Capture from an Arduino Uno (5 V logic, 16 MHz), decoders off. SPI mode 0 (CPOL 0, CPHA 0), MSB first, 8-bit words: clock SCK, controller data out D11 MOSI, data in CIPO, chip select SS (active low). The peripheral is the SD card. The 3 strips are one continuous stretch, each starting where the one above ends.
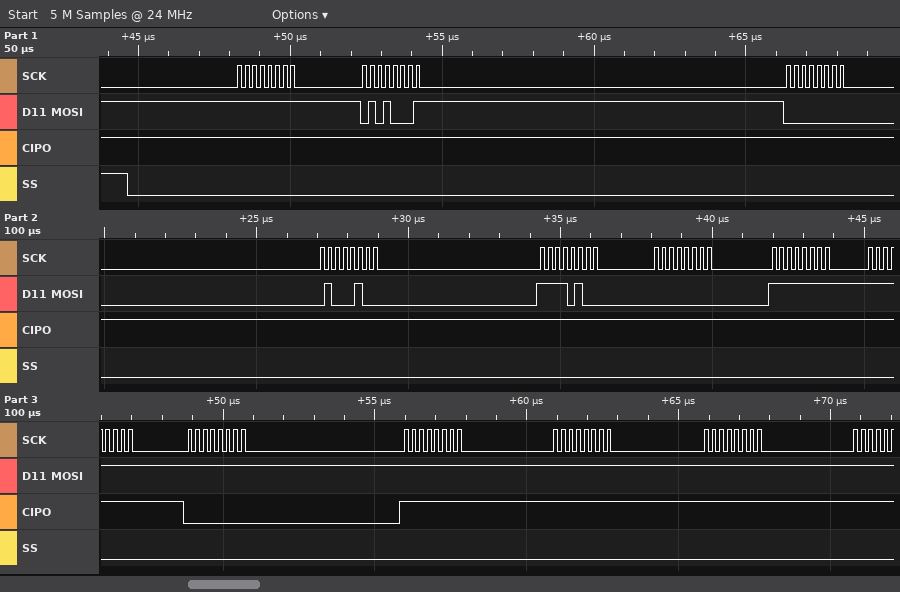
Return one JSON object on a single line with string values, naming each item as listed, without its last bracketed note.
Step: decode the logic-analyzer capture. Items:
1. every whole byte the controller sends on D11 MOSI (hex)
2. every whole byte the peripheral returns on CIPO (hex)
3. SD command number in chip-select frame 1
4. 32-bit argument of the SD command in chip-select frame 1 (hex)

{"every whole byte the controller sends on D11 MOSI": "FF 51 00 44 F4 00 FF FF FF FF FF FF", "every whole byte the peripheral returns on CIPO": "FF FF FF FF FF FF FF FF 00 FF FF FF", "SD command number in chip-select frame 1": "CMD17", "32-bit argument of the SD command in chip-select frame 1": "0x0044F400"}
